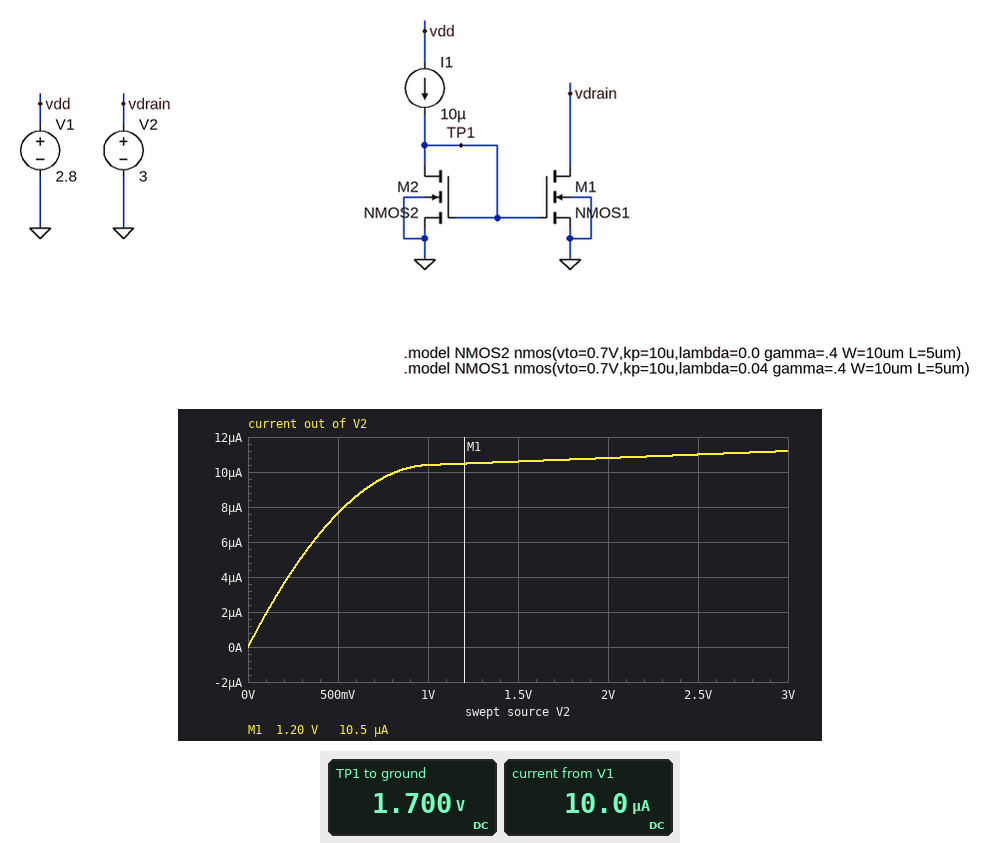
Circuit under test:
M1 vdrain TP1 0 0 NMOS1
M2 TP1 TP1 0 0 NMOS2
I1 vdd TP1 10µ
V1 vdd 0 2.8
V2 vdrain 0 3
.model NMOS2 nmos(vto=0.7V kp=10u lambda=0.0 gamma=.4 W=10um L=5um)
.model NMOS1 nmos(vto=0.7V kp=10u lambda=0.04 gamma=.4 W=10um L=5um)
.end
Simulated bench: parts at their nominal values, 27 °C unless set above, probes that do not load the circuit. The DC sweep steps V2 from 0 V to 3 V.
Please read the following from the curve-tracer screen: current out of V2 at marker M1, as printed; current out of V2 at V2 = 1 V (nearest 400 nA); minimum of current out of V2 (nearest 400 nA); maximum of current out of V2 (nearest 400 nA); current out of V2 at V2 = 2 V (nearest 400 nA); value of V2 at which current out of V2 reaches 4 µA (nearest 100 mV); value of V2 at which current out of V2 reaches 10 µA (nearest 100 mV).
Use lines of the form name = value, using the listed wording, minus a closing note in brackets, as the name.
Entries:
current out of V2 at marker M1, as printed = 10.5 µA
current out of V2 at V2 = 1 V = 10.4 µA
minimum of current out of V2 = 0 A
maximum of current out of V2 = 11.2 µA
current out of V2 at V2 = 2 V = 10.8 µA
value of V2 at which current out of V2 reaches 4 µA = 200 mV
value of V2 at which current out of V2 reaches 10 µA = 800 mV
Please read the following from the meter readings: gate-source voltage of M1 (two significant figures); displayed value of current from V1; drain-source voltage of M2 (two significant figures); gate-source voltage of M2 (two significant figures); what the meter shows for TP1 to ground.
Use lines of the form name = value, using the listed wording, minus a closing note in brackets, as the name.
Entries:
gate-source voltage of M1 = 1.7 V
displayed value of current from V1 = 10.0 µA
drain-source voltage of M2 = 1.7 V
gate-source voltage of M2 = 1.7 V
what the meter shows for TP1 to ground = 1.700 V
